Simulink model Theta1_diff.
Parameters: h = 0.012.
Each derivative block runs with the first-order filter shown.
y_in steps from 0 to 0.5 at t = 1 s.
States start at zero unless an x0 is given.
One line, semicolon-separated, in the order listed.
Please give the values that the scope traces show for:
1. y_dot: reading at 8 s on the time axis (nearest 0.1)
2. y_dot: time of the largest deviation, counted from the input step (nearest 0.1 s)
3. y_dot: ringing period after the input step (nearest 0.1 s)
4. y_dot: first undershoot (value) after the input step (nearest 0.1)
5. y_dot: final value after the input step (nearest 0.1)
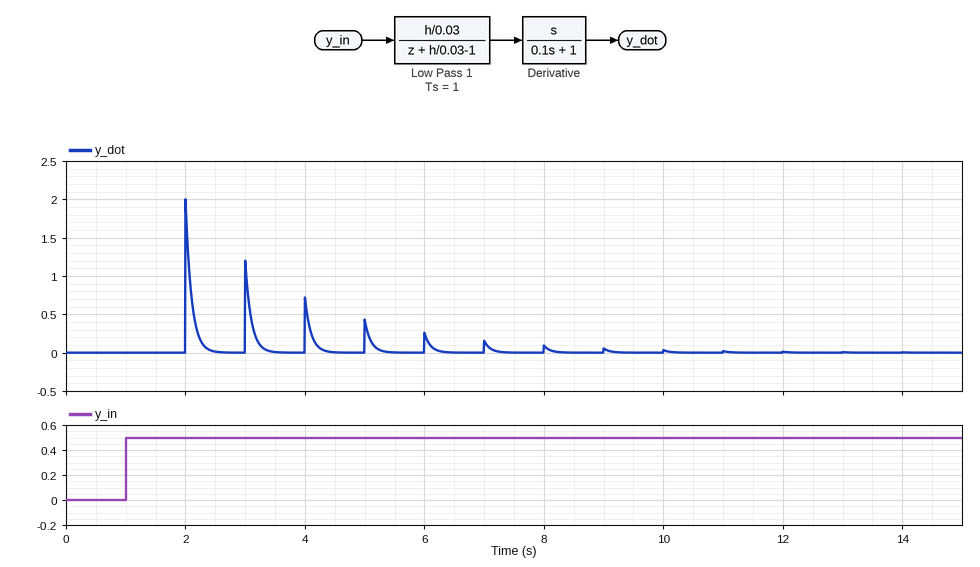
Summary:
0.1; 1.0 s; 1.0 s; 0.0; 0.0
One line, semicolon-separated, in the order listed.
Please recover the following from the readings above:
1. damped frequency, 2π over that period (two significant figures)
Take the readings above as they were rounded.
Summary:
6.3 rad/s
